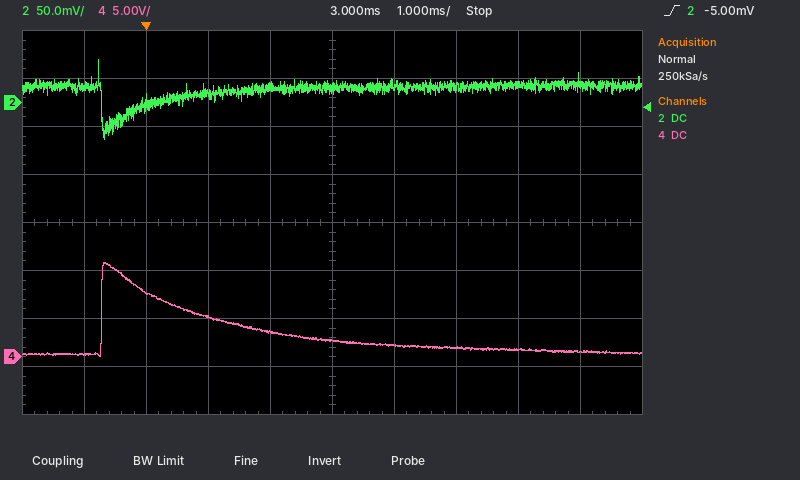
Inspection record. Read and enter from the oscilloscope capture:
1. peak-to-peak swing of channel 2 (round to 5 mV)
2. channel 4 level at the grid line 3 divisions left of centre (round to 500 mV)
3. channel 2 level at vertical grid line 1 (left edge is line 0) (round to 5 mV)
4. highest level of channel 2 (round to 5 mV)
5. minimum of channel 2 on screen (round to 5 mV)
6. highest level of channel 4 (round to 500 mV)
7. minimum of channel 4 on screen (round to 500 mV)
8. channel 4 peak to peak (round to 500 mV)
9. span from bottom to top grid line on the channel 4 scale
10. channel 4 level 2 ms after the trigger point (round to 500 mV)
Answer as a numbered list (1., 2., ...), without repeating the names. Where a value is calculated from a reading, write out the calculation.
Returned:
1. 45 mV − (-40 mV) = 85 mV
2. 6.5 V
3. 15 mV
4. 45 mV
5. -40 mV
6. 10.0 V
7. 0.0 V
8. 10.0 V − (0.0 V) = 10.0 V
9. 40 V
10. 2.5 V
